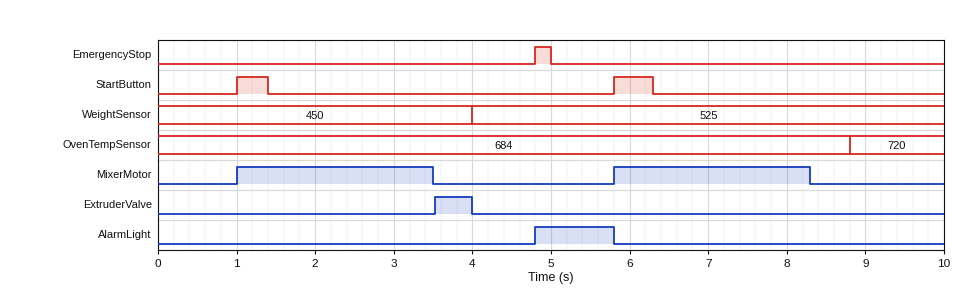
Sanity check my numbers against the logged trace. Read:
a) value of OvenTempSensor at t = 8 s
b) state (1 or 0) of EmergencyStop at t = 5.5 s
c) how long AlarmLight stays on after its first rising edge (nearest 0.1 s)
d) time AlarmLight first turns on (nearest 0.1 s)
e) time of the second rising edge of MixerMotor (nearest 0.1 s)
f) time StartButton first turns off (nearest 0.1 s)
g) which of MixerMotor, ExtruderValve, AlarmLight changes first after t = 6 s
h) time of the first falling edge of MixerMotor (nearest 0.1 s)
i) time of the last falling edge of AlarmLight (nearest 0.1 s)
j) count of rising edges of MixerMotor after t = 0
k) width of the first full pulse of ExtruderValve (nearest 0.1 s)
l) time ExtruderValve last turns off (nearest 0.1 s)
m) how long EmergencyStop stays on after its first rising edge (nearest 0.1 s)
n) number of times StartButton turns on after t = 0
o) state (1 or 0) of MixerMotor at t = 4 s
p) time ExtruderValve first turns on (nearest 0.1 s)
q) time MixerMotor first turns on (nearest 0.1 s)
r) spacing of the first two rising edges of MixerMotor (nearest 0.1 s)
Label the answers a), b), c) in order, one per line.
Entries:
a) 684
b) 0
c) 1.0 s
d) 4.8 s
e) 5.8 s
f) 1.4 s
g) MixerMotor
h) 3.5 s
i) 5.8 s
j) 2
k) 0.5 s
l) 4.0 s
m) 0.2 s
n) 2
o) 0
p) 3.5 s
q) 1.0 s
r) 4.8 s
